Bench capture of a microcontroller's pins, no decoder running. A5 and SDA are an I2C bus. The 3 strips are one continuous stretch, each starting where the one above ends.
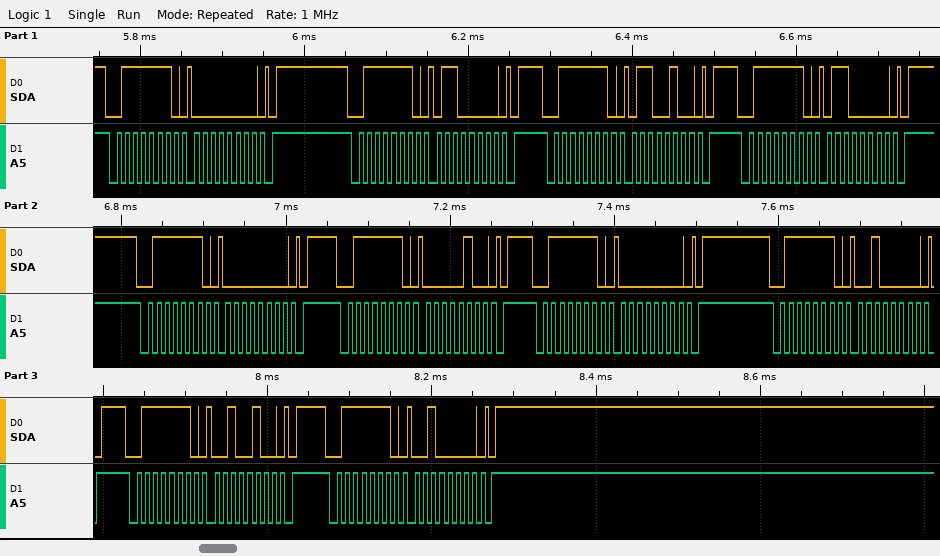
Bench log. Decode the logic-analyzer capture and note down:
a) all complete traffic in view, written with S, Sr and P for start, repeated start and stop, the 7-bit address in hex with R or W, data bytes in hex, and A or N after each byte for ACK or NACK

S 3FW A 00 A P S 3FW A 60 A P S 3FW A 64 A P S 3FW A 60 A P S 3FW A 00 A P S 3FW A 04 A P S 3FW A 00 A P S 3FW A 20 A P S 3FW A 24 A P S 3FW A 20 A P
